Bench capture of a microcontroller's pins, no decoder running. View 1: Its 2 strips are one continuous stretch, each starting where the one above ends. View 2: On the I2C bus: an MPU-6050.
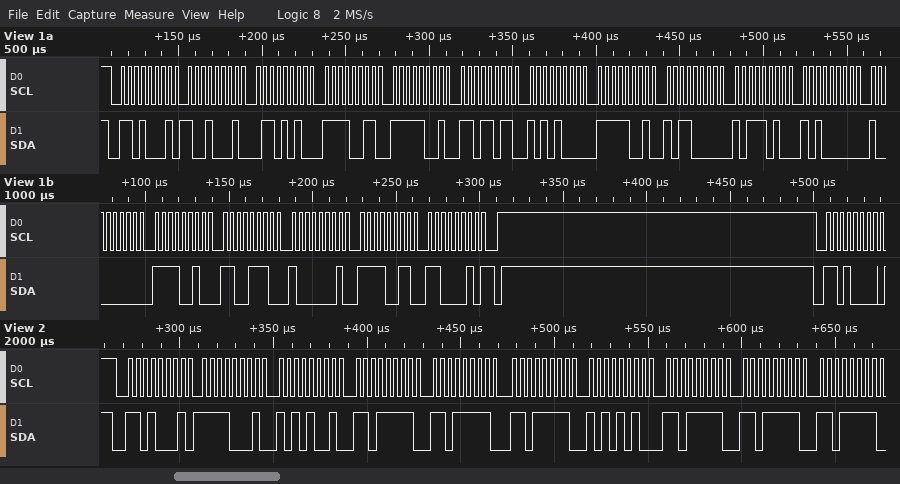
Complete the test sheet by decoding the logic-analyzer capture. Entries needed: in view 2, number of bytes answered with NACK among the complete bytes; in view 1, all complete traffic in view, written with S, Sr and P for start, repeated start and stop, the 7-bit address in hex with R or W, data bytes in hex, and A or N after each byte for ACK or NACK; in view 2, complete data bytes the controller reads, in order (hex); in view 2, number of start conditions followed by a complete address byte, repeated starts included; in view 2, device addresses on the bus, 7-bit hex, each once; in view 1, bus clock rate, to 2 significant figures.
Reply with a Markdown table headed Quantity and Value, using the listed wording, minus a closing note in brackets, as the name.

| Quantity | Value |
|---|---|
| in view 2, number of bytes answered with NACK among the complete bytes | 0 |
| in view 1, all complete traffic in view, written with S, Sr and P for start, repeated start and stop, the 7-bit address in hex with R or W, data bytes in hex, and A or N after each byte for ACK or NACK | S 68R A 91 A 6A A F3 A F9 A DB A A8 A F9 A B0 A BA A A0 A 80 A F2 A CE A 81 A F3 A C2 N P S 68W A |
| in view 2, complete data bytes the controller reads, in order | F1 A9 DF DF DF AA DF DF DF |
| in view 2, number of start conditions followed by a complete address byte, repeated starts included | 1 |
| in view 2, device addresses on the bus, 7-bit hex, each once | 0x68 |
| in view 1, bus clock rate, to 2 significant figures | 250 kHz |
